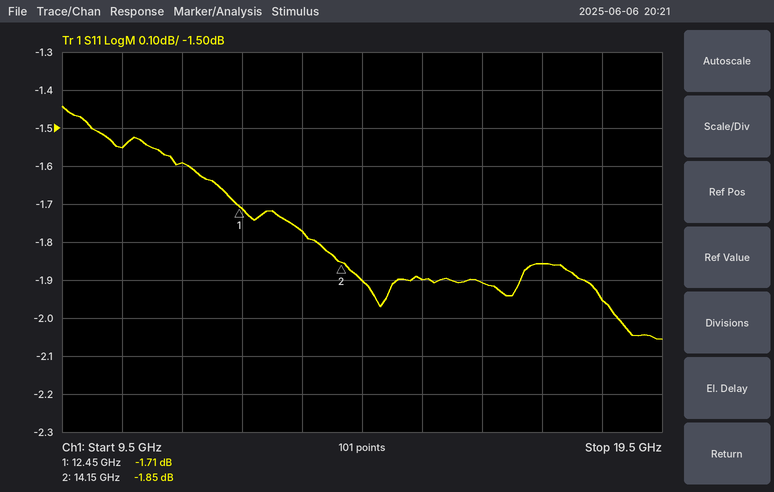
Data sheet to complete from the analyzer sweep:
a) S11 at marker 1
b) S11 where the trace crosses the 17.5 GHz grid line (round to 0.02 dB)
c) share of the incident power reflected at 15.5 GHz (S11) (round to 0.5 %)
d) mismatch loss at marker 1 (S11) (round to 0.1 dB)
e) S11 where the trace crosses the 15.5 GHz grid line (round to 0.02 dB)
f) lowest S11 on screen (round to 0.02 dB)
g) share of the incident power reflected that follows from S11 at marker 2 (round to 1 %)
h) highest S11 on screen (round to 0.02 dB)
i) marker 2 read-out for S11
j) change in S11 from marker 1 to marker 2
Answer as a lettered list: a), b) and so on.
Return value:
a) -1.71 dB
b) -1.86 dB
c) 64.5 %
d) 4.9 dB
e) -1.90 dB
f) -2.06 dB
g) 65 %
h) -1.44 dB
i) -1.85 dB
j) -0.14 dB
